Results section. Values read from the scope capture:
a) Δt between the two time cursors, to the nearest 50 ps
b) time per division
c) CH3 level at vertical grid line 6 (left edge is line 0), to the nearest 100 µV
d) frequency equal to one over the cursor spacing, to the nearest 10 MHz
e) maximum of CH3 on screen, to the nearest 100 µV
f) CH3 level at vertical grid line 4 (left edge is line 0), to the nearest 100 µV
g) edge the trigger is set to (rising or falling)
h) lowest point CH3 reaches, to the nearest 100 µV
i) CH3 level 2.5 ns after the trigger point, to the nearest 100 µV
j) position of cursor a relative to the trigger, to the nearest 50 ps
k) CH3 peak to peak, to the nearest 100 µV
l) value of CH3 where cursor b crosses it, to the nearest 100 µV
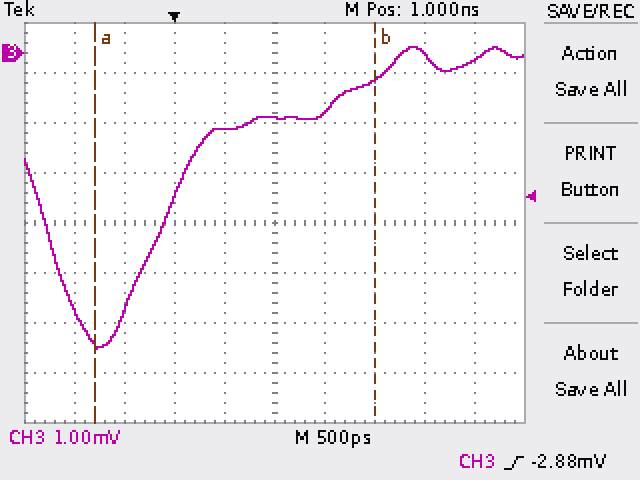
2.80 ns
500 ps
-1.2 mV
360 MHz
100 µV
-1.5 mV
rising
-5.9 mV
0.0 mV
-800 ps
6.0 mV
-500 µV
